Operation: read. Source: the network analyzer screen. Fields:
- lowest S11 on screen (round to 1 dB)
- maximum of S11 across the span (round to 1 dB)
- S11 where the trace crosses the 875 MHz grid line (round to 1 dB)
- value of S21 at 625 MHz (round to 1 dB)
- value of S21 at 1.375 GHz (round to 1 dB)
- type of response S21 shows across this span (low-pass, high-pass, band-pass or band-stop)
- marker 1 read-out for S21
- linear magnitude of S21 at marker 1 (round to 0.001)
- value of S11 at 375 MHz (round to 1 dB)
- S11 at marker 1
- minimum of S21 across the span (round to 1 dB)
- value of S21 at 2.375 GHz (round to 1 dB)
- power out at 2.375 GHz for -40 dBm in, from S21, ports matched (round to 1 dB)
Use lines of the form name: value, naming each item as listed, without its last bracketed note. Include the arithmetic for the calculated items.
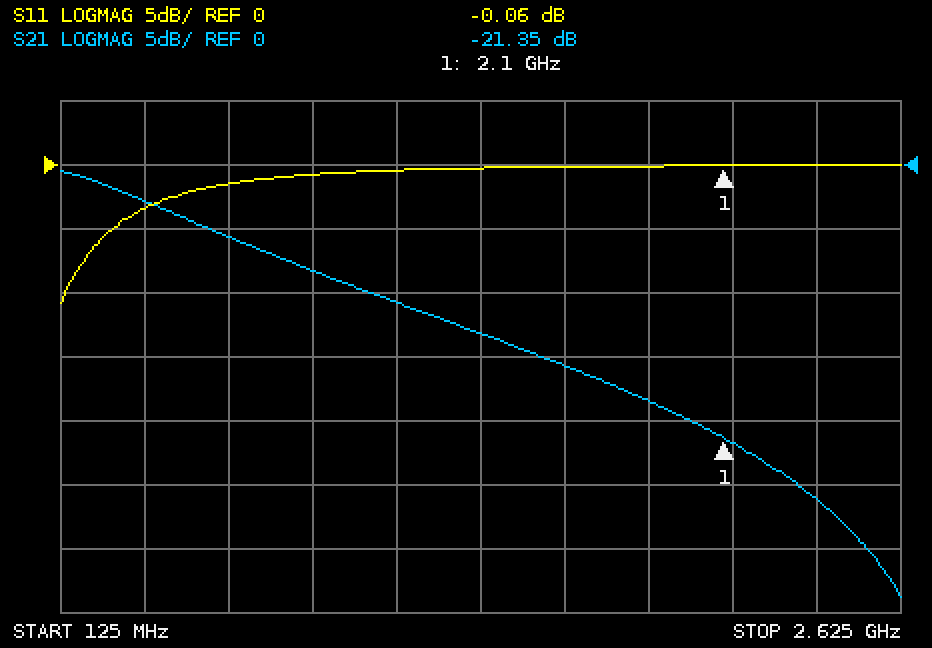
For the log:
lowest S11 on screen: -11 dB
maximum of S11 across the span: 0 dB
S11 where the trace crosses the 875 MHz grid line: -1 dB
value of S21 at 625 MHz: -6 dB
value of S21 at 1.375 GHz: -13 dB
type of response S21 shows across this span: low-pass
marker 1 read-out for S21: -21.35 dB
linear magnitude of S21 at marker 1: 10^(-21.35/20) ≈ 0.086
value of S11 at 375 MHz: -3 dB
S11 at marker 1: -0.06 dB
minimum of S21 across the span: -34 dB
value of S21 at 2.375 GHz: -26 dB
power out at 2.375 GHz for -40 dBm in, from S21, ports matched: -40 dBm + (-26 dB) = -66 dBm
